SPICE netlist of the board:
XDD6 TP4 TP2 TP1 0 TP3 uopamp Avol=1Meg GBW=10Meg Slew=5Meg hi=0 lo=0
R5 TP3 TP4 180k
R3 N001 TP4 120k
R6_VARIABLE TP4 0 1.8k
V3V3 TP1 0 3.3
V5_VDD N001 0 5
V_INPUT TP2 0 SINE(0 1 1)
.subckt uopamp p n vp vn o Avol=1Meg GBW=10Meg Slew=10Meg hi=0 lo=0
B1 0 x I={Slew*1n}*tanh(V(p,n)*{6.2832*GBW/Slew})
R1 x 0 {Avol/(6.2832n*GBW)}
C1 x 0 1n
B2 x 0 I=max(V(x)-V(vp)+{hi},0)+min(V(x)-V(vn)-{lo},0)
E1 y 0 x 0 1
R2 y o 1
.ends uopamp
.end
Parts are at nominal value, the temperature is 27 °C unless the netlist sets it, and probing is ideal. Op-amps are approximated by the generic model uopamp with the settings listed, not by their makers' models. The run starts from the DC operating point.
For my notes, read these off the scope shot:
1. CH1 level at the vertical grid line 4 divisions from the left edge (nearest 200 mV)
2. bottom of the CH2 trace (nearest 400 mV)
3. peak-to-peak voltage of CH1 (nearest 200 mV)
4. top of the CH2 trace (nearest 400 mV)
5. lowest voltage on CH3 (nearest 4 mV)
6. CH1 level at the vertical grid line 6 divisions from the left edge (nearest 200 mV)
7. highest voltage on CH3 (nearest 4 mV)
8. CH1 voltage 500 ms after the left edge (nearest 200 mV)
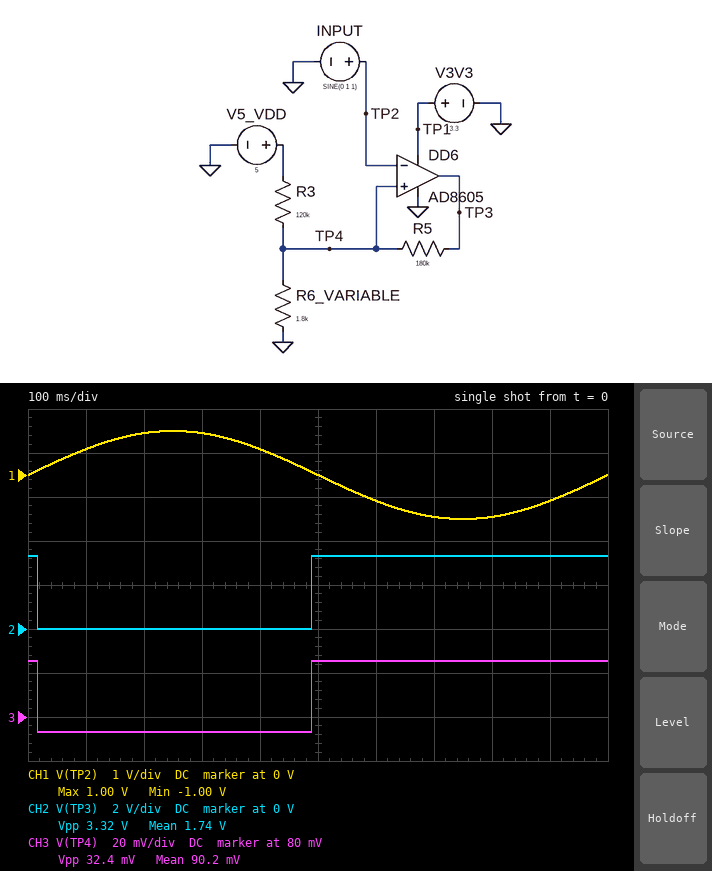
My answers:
600 mV
0 V
2.0 V
3.2 V
72 mV
-600 mV
104 mV
0 V
